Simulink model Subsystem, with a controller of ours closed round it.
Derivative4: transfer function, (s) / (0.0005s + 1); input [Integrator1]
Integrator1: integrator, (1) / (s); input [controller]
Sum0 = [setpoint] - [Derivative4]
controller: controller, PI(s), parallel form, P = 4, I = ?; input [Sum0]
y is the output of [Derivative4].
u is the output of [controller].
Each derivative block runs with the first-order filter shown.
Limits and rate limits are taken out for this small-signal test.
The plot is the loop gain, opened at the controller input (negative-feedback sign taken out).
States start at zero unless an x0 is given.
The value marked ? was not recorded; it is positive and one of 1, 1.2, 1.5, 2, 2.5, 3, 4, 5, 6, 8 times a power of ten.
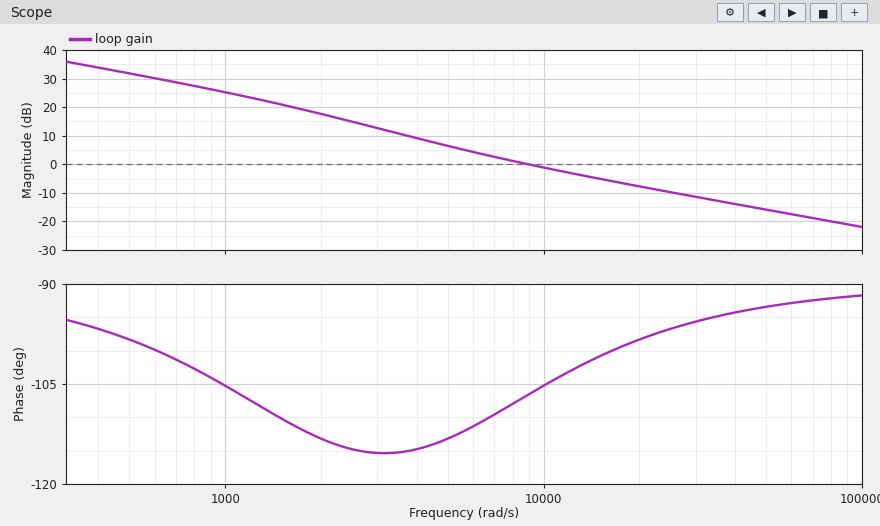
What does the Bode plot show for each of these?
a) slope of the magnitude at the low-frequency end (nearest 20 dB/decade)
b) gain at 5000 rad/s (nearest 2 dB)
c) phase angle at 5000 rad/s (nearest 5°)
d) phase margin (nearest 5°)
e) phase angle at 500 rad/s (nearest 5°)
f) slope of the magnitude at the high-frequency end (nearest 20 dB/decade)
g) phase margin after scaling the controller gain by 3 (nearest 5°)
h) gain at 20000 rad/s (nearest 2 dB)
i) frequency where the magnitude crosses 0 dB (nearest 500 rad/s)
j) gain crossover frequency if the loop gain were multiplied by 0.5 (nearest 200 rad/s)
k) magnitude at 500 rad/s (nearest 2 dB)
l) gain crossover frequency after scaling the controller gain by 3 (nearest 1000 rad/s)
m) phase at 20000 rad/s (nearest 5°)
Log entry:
-20 dB/decade
6 dB
-115°
75°
-100°
-20 dB/decade
85°
-8 dB
9000 rad/s
5200 rad/s
32 dB
24000 rad/s
-100°
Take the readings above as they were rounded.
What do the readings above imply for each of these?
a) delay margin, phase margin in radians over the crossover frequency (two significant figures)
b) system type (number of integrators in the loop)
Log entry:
0.00015 s
1
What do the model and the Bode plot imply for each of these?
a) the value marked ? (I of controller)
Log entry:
20000
